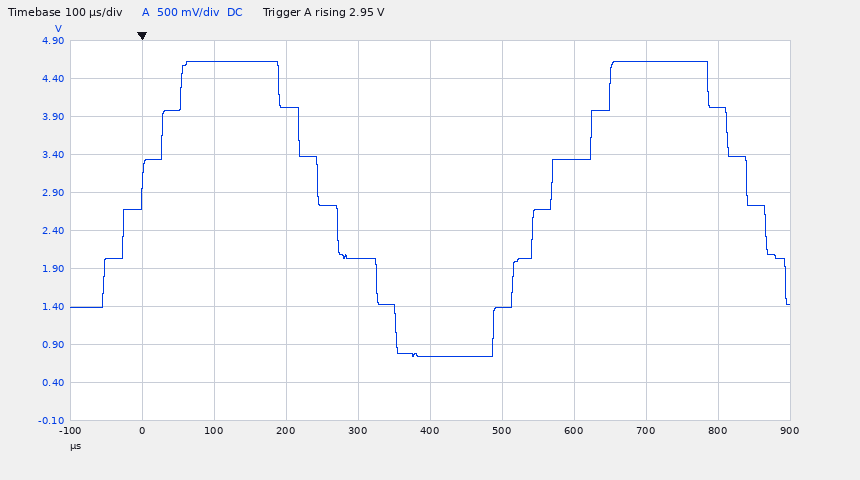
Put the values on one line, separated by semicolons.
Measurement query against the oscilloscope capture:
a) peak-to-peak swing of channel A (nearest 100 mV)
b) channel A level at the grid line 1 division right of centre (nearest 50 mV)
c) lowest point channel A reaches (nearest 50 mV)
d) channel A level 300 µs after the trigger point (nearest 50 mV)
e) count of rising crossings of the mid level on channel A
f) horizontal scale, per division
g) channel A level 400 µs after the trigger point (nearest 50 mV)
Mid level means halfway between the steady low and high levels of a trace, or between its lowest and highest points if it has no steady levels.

3.90 V; 1.40 V; 750 mV; 2.05 V; 2; 100 µs; 750 mV
